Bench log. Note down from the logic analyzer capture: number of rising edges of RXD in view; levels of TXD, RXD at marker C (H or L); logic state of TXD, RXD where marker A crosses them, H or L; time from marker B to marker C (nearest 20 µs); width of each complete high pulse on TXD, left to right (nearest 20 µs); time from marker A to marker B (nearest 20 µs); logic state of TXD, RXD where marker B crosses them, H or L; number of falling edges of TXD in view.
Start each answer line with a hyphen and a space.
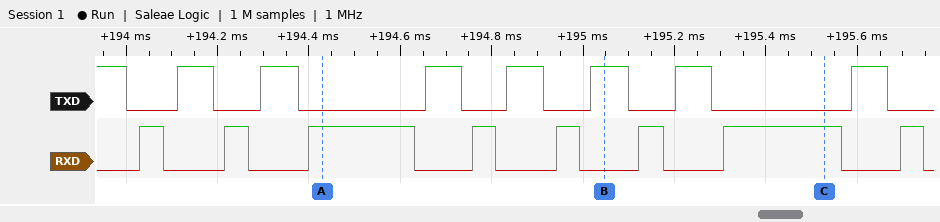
- 8
- TXD=L, RXD=H
- TXD=L, RXD=H
- 480 µs
- 80 µs, 80 µs, 80 µs, 80 µs, 80 µs, 80 µs, 80 µs
- 620 µs
- TXD=H, RXD=L
- 8
